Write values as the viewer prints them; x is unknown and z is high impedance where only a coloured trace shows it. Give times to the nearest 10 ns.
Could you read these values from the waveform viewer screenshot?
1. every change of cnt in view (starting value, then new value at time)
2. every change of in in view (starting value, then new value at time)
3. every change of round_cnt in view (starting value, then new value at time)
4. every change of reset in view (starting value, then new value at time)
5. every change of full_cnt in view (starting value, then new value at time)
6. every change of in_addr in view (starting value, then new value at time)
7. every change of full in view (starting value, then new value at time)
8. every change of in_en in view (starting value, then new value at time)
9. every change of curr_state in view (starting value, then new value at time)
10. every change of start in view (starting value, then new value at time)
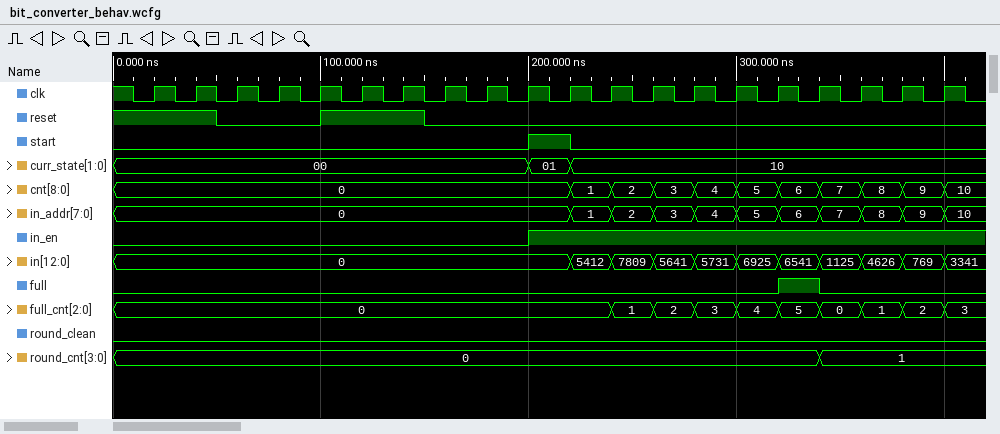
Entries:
0, 1 at 220 ns, 2 at 240 ns, 3 at 260 ns, 4 at 280 ns, 5 at 300 ns, 6 at 320 ns, 7 at 340 ns, 8 at 360 ns, 9 at 380 ns, 10 at 400 ns
0, 5412 at 220 ns, 7809 at 240 ns, 5641 at 260 ns, 5731 at 280 ns, 6925 at 300 ns, 6541 at 320 ns, 1125 at 340 ns, 4626 at 360 ns, 769 at 380 ns, 3341 at 400 ns
0, 1 at 340 ns
1, 0 at 50 ns, 1 at 100 ns, 0 at 150 ns
0, 1 at 240 ns, 2 at 260 ns, 3 at 280 ns, 4 at 300 ns, 5 at 320 ns, 0 at 340 ns, 1 at 360 ns, 2 at 380 ns, 3 at 400 ns
0, 1 at 220 ns, 2 at 240 ns, 3 at 260 ns, 4 at 280 ns, 5 at 300 ns, 6 at 320 ns, 7 at 340 ns, 8 at 360 ns, 9 at 380 ns, 10 at 400 ns
0, 1 at 320 ns, 0 at 340 ns
0, 1 at 200 ns
00, 01 at 200 ns, 10 at 220 ns
0, 1 at 200 ns, 0 at 220 ns
